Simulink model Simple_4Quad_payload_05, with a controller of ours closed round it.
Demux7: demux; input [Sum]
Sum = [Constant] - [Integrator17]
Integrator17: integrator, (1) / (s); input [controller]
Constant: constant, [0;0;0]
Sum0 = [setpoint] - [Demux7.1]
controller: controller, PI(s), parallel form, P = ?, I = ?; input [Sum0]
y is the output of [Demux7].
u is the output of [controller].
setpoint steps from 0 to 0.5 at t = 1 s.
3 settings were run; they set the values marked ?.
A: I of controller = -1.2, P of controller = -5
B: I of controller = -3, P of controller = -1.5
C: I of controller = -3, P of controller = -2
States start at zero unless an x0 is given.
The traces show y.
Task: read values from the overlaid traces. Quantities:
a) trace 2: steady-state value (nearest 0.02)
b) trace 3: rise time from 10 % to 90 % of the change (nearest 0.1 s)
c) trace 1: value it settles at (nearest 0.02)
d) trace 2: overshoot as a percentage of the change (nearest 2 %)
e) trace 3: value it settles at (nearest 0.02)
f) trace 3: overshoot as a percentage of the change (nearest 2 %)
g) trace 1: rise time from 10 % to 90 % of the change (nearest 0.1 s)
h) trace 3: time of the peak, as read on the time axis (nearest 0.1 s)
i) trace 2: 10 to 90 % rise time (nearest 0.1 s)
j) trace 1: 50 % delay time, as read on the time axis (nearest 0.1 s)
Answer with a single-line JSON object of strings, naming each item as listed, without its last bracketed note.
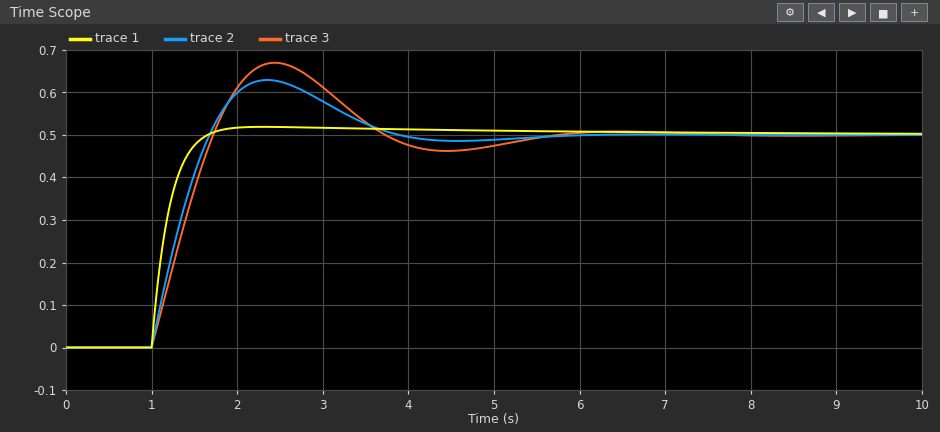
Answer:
{"trace 2: steady-state value": "0.50", "trace 3: rise time from 10 % to 90 % of the change": "0.6 s", "trace 1: value it settles at": "0.50", "trace 2: overshoot as a percentage of the change": "26 %", "trace 3: value it settles at": "0.50", "trace 3: overshoot as a percentage of the change": "34 %", "trace 1: rise time from 10 % to 90 % of the change": "0.4 s", "trace 3: time of the peak, as read on the time axis": "2.4 s", "trace 2: 10 to 90 % rise time": "0.5 s", "trace 1: 50 % delay time, as read on the time axis": "1.1 s"}
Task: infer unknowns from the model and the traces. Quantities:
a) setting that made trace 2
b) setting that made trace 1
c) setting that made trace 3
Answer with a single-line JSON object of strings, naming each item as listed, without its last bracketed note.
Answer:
{"setting that made trace 2": "C", "setting that made trace 1": "A", "setting that made trace 3": "B"}
